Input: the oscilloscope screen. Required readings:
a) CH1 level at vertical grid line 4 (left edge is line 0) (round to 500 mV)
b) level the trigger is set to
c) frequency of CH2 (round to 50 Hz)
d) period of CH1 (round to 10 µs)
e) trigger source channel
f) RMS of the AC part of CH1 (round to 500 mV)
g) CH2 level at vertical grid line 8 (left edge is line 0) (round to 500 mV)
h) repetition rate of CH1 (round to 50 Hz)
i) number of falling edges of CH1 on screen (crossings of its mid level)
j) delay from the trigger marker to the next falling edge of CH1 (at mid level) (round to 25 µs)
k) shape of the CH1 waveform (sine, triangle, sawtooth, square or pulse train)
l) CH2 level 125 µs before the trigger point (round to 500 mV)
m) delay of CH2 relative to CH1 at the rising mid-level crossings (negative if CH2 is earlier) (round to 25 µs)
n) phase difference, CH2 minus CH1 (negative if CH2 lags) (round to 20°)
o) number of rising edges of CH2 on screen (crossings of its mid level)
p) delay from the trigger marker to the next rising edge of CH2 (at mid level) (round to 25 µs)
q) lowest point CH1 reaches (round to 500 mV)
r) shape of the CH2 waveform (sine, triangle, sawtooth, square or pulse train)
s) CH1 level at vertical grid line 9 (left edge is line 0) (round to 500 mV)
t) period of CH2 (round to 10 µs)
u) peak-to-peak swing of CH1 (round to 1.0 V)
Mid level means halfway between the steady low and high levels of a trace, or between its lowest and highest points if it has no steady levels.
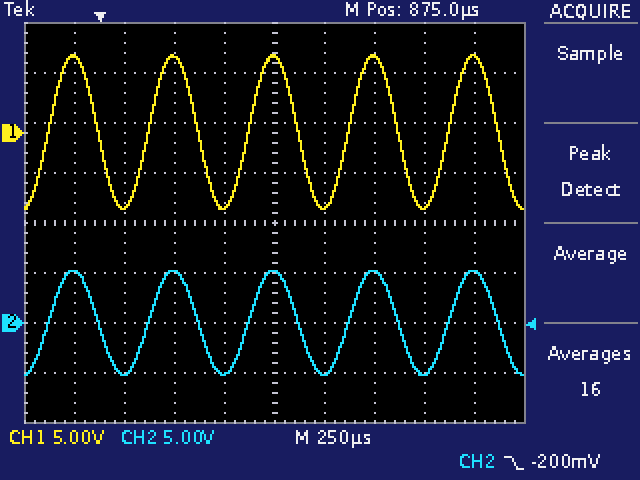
-7.5 V
-200 mV
2.00 kHz
500 µs
CH2
5.5 V
-5.0 V
2.00 kHz
5
500 µs
sine
5.0 V
0 µs
0°
5
250 µs
-7.5 V
sine
7.5 V
500 µs
15.0 V
